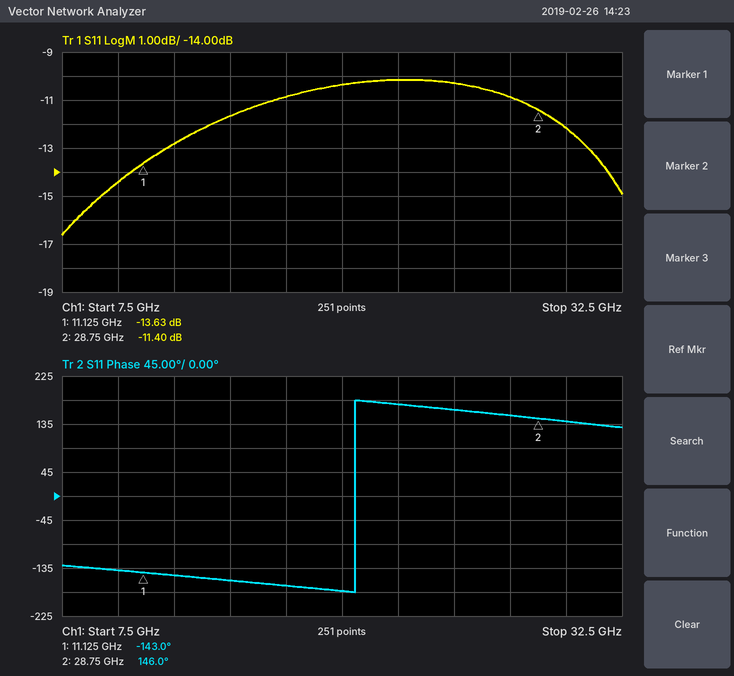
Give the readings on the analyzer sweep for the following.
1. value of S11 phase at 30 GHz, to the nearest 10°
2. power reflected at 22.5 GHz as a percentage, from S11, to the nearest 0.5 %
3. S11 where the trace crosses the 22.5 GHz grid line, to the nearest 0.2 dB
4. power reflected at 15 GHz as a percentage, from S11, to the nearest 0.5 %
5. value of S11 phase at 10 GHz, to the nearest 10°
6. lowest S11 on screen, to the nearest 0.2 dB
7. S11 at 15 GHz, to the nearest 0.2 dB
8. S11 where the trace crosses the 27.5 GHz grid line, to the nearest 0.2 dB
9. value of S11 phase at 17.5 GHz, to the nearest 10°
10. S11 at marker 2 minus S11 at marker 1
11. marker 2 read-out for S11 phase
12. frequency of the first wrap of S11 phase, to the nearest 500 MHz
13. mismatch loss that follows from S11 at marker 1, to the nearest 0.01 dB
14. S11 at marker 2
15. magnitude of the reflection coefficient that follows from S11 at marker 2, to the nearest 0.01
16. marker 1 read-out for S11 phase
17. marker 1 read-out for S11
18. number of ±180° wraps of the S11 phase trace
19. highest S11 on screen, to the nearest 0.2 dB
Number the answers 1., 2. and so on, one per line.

1. 140°
2. 9.5 %
3. -10.2 dB
4. 7.0 %
5. -140°
6. -16.6 dB
7. -11.6 dB
8. -10.8 dB
9. -170°
10. 2.23 dB
11. 146.0°
12. 20.5 GHz
13. 0.19 dB
14. -11.40 dB
15. 0.27
16. -143.0°
17. -13.63 dB
18. 1
19. -10.2 dB
